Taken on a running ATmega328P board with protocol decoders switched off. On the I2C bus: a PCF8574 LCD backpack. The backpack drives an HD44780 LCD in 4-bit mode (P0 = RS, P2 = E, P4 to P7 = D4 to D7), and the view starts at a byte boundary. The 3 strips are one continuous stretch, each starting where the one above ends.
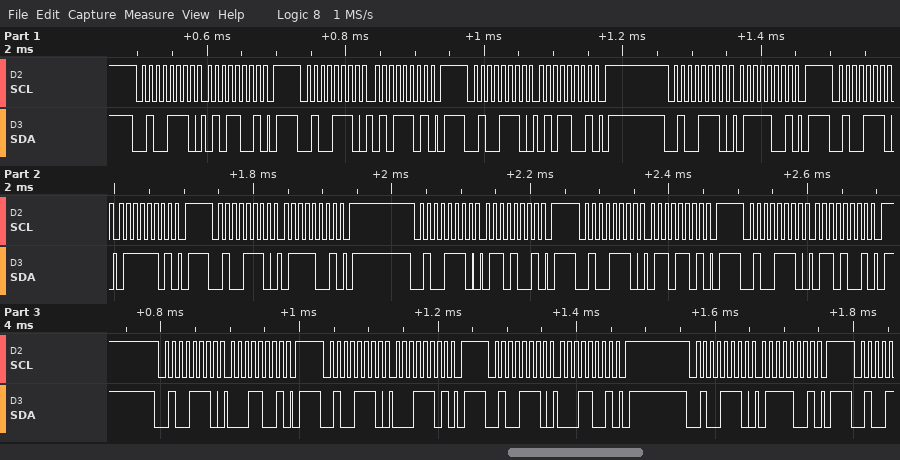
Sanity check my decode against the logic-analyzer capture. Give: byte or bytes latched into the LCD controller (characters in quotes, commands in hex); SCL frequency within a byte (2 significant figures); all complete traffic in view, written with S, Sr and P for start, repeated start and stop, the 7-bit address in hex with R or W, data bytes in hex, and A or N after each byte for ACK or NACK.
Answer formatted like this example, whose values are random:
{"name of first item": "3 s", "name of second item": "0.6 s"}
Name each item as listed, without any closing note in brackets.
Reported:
{"byte or bytes latched into the LCD controller": "'W' 'a'", "SCL frequency within a byte": "100 kHz", "all complete traffic in view, written with S, Sr and P for start, repeated start and stop, the 7-bit address in hex with R or W, data bytes in hex, and A or N after each byte for ACK or NACK": "S 27W A 59 A P S 27W A 5D A P S 27W A 59 A P S 27W A 79 A P S 27W A 7D A P S 27W A 79 A P S 27W A 69 A P S 27W A 6D A P S 27W A 69 A P S 27W A 19 A P S 27W A 1D A P S 27W A 19 A P S 27W A 79 A P"}
